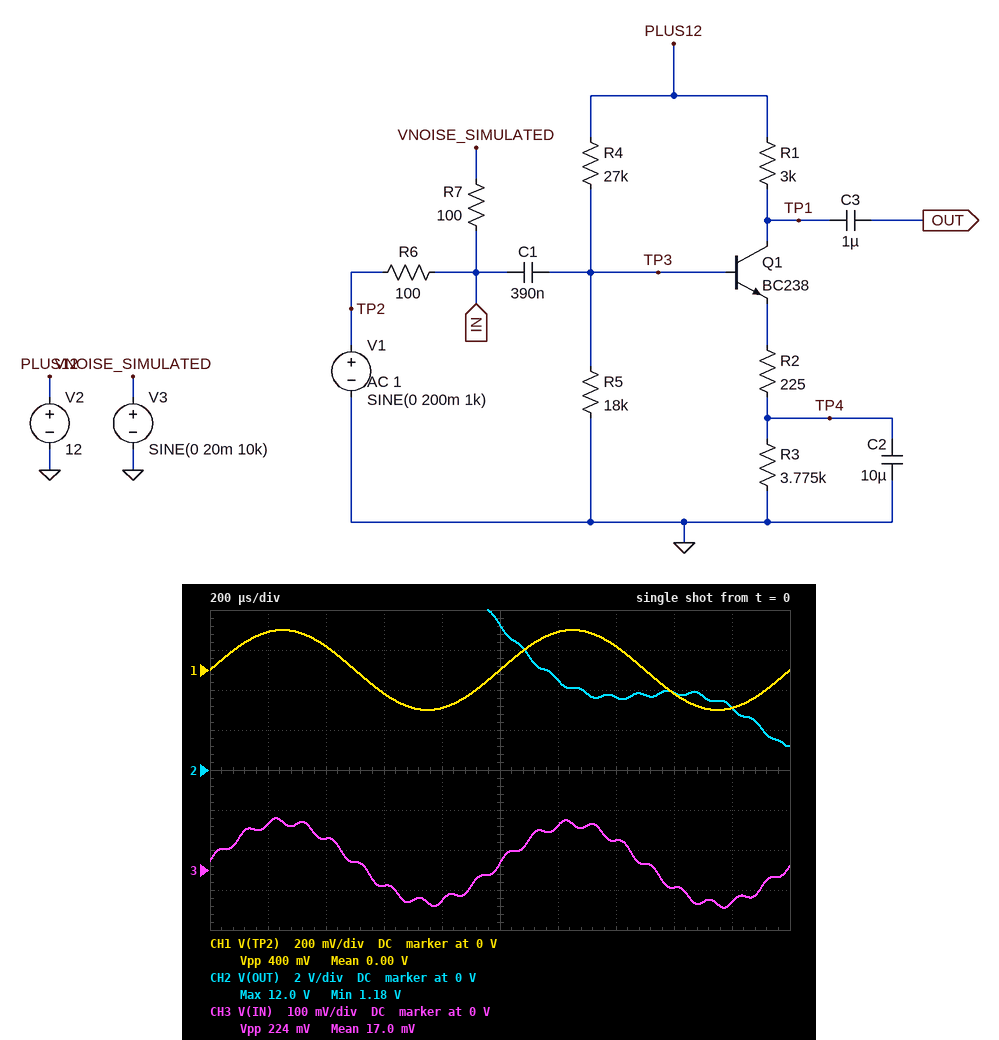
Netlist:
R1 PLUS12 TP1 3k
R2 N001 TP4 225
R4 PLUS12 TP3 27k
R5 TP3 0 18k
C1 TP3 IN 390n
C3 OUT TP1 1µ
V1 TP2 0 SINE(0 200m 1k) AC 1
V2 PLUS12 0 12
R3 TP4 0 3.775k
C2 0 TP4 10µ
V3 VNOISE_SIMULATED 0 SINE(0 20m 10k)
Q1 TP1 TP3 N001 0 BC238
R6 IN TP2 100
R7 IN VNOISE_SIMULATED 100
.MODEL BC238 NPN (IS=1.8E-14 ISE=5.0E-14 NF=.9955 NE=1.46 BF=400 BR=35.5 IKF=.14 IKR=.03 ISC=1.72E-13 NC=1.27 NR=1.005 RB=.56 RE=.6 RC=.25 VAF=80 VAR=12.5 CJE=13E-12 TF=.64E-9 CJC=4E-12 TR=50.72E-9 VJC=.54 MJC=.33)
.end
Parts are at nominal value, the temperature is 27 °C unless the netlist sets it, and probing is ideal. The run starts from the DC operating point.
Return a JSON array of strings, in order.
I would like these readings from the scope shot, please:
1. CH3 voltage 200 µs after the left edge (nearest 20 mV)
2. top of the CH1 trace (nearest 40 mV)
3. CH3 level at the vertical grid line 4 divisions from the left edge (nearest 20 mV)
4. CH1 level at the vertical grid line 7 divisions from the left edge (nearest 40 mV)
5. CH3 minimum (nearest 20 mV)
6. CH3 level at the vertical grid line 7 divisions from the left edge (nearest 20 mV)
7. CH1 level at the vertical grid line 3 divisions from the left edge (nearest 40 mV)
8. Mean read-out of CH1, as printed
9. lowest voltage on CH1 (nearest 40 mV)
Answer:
["120 mV", "200 mV", "-80 mV", "120 mV", "-100 mV", "80 mV", "-120 mV", "0.00 V", "-200 mV"]
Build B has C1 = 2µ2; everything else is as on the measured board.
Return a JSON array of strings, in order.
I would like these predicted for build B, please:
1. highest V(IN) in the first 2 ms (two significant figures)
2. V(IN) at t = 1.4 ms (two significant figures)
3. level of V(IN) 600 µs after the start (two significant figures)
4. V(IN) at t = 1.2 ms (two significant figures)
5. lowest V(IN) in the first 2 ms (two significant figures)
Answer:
["130 mV", "79 mV", "-37 mV", "120 mV", "-88 mV"]
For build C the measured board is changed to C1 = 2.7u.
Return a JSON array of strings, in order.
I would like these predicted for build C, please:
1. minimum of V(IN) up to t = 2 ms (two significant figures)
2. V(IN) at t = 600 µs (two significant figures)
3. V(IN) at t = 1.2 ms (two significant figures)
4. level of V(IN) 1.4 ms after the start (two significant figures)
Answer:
["-88 mV", "-37 mV", "120 mV", "80 mV"]
